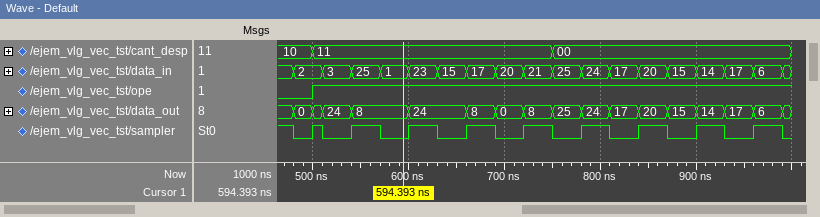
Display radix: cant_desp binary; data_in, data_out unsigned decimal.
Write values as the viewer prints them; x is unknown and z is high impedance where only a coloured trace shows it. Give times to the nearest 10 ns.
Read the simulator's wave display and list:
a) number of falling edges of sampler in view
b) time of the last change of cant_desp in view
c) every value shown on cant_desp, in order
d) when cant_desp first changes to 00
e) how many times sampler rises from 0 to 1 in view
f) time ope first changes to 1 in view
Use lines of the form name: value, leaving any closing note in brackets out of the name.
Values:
number of falling edges of sampler in view: 10
time of the last change of cant_desp in view: 750 ns
every value shown on cant_desp, in order: 10, 11, 00
when cant_desp first changes to 00: 750 ns
how many times sampler rises from 0 to 1 in view: 9
time ope first changes to 1 in view: 500 ns
